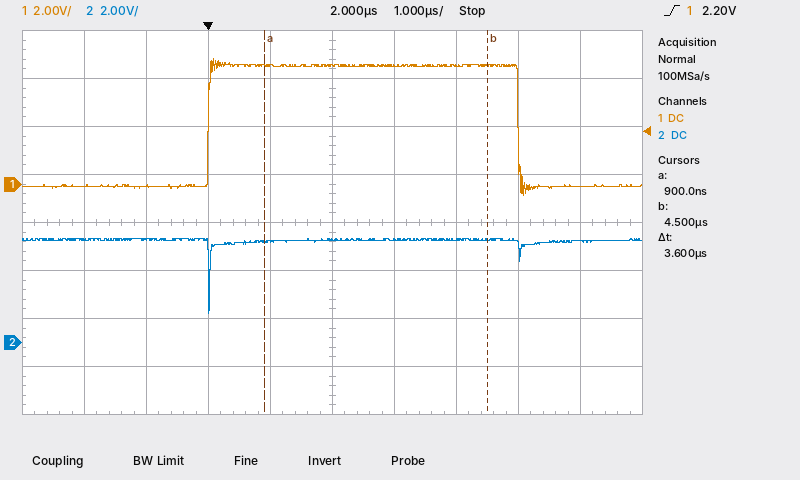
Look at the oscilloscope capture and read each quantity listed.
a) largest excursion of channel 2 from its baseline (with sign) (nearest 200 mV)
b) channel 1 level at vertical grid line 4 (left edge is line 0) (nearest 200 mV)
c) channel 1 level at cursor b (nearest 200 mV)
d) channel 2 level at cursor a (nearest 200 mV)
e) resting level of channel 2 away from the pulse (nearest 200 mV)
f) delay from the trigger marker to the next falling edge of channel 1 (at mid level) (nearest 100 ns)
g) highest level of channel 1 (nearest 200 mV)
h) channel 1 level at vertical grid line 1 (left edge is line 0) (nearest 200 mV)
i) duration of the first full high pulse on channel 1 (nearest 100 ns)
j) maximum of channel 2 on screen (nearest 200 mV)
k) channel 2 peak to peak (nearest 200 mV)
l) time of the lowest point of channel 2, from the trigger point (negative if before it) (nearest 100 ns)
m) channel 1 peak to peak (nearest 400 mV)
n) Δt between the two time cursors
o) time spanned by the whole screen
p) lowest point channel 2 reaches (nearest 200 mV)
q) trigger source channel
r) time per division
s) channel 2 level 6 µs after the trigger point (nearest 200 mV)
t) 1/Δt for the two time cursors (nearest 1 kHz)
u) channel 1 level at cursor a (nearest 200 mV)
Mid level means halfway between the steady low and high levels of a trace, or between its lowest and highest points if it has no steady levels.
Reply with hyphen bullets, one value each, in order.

- -3.0 V
- 5.0 V
- 5.0 V
- 4.2 V
- 4.2 V
- 5.0 µs
- 5.2 V
- 0.0 V
- 5.0 µs
- 4.4 V
- 3.2 V
- 0.0 µs
- 5.6 V
- 3.6 µs
- 10 µs
- 1.2 V
- channel 1
- 1 µs
- 4.2 V
- 278 kHz
- 5.0 V
